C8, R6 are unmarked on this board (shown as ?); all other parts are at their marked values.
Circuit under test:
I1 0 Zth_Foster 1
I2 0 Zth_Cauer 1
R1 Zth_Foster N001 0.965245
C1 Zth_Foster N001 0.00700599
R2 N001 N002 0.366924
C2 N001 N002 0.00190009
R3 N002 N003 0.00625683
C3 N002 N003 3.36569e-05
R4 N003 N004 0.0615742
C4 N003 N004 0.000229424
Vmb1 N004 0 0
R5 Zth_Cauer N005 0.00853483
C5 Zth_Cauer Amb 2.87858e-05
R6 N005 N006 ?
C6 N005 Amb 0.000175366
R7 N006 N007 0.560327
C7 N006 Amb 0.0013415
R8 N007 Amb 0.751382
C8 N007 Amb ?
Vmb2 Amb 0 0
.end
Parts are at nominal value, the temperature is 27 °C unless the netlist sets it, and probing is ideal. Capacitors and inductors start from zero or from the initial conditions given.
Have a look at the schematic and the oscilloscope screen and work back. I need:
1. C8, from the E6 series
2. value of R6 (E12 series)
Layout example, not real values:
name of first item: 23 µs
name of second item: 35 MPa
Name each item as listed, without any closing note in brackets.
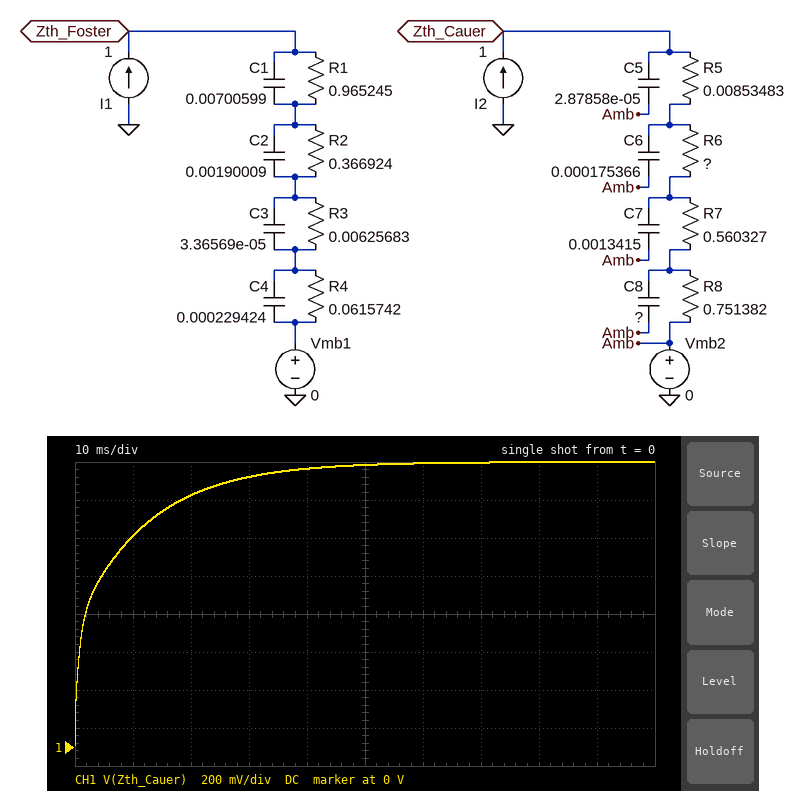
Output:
C8, from the E6 series: 15 mF
value of R6: 0.18 Ω
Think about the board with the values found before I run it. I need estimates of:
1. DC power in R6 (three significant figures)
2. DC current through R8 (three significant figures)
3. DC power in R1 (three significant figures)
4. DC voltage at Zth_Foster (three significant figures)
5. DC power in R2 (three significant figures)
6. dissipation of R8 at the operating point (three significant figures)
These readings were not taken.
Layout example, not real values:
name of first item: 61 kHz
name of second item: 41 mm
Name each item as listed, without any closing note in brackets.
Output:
DC power in R6: 180 mW
DC current through R8: 1.00 A
DC power in R1: 965 mW
DC voltage at Zth_Foster: 1.40 V
DC power in R2: 367 mW
dissipation of R8 at the operating point: 751 mW
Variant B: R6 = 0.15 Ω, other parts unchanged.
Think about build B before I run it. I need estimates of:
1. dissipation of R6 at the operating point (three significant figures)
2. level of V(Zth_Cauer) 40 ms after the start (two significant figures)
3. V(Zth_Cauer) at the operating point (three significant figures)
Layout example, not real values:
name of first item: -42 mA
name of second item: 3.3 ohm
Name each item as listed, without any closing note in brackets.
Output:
dissipation of R6 at the operating point: 150 mW
level of V(Zth_Cauer) 40 ms after the start: 1.4 V
V(Zth_Cauer) at the operating point: 1.47 V
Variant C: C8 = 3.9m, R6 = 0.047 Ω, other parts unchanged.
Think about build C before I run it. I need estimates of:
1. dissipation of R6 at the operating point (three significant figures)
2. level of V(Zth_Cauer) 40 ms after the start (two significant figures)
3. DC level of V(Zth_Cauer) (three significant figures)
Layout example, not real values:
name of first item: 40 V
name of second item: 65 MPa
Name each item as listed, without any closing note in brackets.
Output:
dissipation of R6 at the operating point: 47.0 mW
level of V(Zth_Cauer) 40 ms after the start: 1.4 V
DC level of V(Zth_Cauer): 1.37 V
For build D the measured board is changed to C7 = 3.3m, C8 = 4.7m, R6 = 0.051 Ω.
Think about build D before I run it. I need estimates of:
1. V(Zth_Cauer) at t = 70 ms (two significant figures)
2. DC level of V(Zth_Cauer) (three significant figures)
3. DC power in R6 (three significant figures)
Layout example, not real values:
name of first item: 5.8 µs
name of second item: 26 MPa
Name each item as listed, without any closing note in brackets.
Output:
V(Zth_Cauer) at t = 70 ms: 1.4 V
DC level of V(Zth_Cauer): 1.37 V
DC power in R6: 51.0 mW
